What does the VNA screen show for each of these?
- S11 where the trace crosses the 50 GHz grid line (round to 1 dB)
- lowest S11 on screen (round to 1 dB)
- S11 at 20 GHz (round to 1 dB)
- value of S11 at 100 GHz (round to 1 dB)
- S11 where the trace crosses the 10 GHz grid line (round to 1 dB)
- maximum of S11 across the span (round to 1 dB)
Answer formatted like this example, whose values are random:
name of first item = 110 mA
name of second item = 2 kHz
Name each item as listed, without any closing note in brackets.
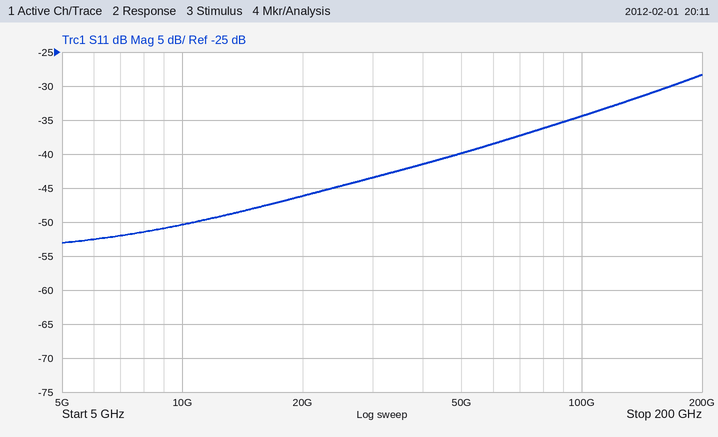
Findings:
S11 where the trace crosses the 50 GHz grid line = -40 dB
lowest S11 on screen = -53 dB
S11 at 20 GHz = -46 dB
value of S11 at 100 GHz = -34 dB
S11 where the trace crosses the 10 GHz grid line = -50 dB
maximum of S11 across the span = -28 dB
